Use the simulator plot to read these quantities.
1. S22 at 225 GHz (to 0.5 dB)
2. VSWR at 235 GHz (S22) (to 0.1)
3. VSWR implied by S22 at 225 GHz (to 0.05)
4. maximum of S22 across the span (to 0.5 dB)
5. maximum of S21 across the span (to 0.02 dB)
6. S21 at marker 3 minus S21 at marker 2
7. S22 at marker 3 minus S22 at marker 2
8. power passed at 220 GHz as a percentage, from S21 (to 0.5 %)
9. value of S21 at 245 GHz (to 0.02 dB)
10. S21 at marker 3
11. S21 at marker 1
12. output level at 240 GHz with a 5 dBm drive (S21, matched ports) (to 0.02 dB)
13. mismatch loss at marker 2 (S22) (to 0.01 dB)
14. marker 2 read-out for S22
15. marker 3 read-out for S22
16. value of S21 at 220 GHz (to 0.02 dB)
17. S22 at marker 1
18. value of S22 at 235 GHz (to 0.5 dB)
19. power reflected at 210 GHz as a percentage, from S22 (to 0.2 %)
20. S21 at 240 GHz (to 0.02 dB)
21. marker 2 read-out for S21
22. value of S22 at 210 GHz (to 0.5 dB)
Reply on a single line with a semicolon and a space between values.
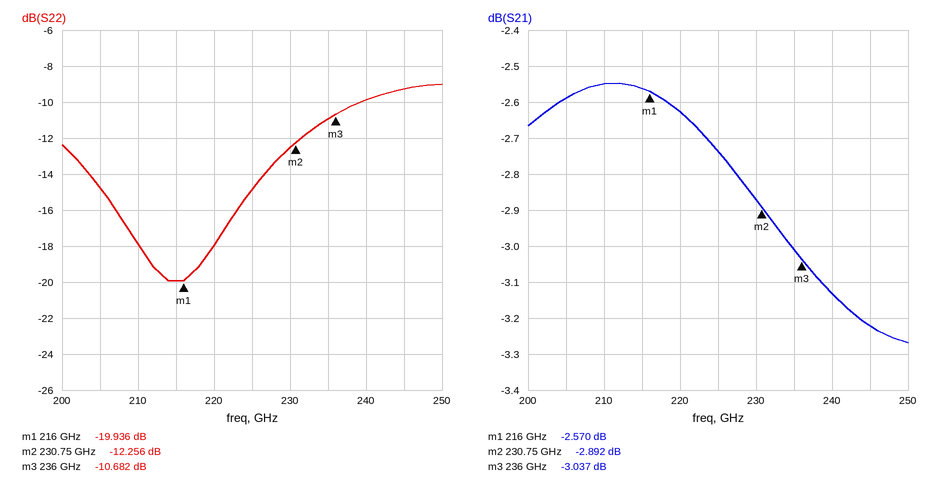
-15.0 dB; 1.8; 1.45; -9.0 dB; -2.54 dB; -0.145 dB; 1.574 dB; 54.5 %; -3.22 dB; -3.037 dB; -2.570 dB; 1.86 dBm; 0.27 dB; -12.256 dB; -10.682 dB; -2.62 dB; -19.936 dB; -11.0 dB; 1.6 %; -3.14 dB; -2.892 dB; -18.0 dB
